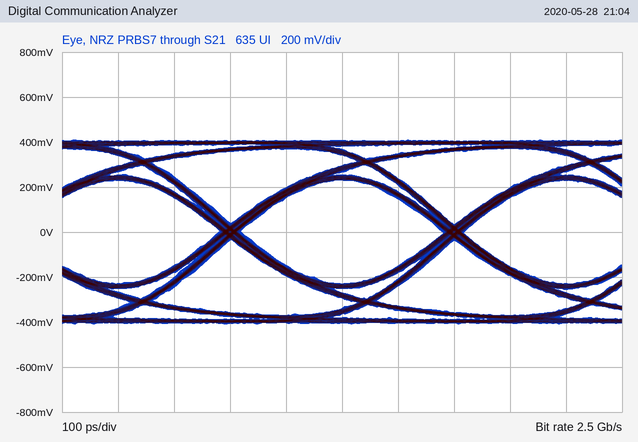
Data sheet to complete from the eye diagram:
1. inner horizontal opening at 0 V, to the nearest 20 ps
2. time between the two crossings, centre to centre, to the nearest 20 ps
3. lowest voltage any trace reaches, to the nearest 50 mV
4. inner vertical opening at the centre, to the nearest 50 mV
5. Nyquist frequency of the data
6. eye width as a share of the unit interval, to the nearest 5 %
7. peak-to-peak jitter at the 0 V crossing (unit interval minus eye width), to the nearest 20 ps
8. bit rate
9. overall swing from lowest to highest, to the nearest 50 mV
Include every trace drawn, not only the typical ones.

360 ps
400 ps
-400 mV
450 mV
1.25 GHz
90 %
40 ps
2.5 Gb/s
800 mV
